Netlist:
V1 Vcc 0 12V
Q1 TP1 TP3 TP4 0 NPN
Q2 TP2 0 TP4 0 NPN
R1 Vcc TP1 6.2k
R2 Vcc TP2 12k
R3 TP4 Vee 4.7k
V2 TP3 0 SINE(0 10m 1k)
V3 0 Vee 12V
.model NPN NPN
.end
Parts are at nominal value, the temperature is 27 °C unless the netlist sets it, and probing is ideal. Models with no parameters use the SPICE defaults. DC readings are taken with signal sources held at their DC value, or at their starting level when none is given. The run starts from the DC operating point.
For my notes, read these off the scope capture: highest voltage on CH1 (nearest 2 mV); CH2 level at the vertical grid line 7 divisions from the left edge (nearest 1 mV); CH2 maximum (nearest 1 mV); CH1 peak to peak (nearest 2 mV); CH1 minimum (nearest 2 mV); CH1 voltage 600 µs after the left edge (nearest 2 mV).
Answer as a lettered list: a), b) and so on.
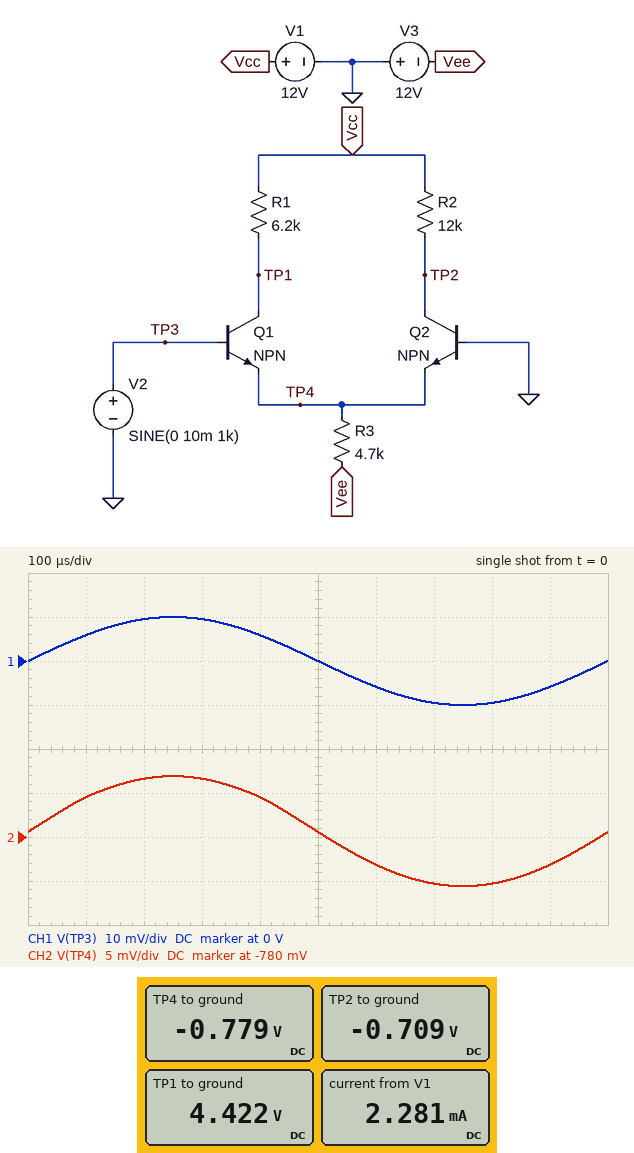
a) 10 mV
b) -785 mV
c) -773 mV
d) 20 mV
e) -10 mV
f) -6 mV
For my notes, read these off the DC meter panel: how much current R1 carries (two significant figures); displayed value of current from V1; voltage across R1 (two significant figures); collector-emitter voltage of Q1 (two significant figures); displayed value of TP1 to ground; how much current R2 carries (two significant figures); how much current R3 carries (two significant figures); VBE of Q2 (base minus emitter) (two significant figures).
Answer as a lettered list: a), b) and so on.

a) 1.2 mA
b) 2.281 mA
c) 7.6 V
d) 5.2 V
e) 4.422 V
f) 1.1 mA
g) 2.4 mA
h) 780 mV
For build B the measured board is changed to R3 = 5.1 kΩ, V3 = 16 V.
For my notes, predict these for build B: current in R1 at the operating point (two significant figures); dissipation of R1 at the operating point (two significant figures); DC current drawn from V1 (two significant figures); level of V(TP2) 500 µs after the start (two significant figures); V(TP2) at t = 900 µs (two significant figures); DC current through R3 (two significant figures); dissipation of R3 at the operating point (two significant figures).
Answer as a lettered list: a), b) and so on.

a) 1.6 mA
b) 16 mW
c) 2.7 mA
d) -740 mV
e) -750 mV
f) 3.0 mA
g) 45 mW
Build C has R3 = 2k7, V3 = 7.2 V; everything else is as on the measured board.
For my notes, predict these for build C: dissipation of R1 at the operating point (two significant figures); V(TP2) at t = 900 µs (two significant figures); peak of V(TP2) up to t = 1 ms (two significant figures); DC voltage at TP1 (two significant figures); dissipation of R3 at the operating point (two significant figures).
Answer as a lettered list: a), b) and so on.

a) 9.2 mW
b) -730 mV
c) 560 mV
d) 4.5 V
e) 15 mW
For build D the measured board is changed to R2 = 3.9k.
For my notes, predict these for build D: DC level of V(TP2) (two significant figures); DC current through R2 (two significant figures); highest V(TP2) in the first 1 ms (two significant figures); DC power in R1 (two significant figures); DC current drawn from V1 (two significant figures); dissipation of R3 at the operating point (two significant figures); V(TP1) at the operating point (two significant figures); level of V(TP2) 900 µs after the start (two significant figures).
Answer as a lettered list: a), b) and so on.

a) 7.4 V
b) 1.2 mA
c) 8.3 V
d) 8.7 mW
e) 2.4 mA
f) 27 mW
g) 4.7 V
h) 6.9 V
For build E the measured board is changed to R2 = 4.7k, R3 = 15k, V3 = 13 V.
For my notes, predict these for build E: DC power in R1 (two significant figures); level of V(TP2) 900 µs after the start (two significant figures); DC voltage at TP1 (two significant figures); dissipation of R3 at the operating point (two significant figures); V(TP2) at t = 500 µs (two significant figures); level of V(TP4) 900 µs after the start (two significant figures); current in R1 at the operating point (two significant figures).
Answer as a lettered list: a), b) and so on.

a) 1.0 mW
b) 9.9 V
c) 9.5 V
d) 10 mW
e) 10 V
f) -750 mV
g) 400 µA
